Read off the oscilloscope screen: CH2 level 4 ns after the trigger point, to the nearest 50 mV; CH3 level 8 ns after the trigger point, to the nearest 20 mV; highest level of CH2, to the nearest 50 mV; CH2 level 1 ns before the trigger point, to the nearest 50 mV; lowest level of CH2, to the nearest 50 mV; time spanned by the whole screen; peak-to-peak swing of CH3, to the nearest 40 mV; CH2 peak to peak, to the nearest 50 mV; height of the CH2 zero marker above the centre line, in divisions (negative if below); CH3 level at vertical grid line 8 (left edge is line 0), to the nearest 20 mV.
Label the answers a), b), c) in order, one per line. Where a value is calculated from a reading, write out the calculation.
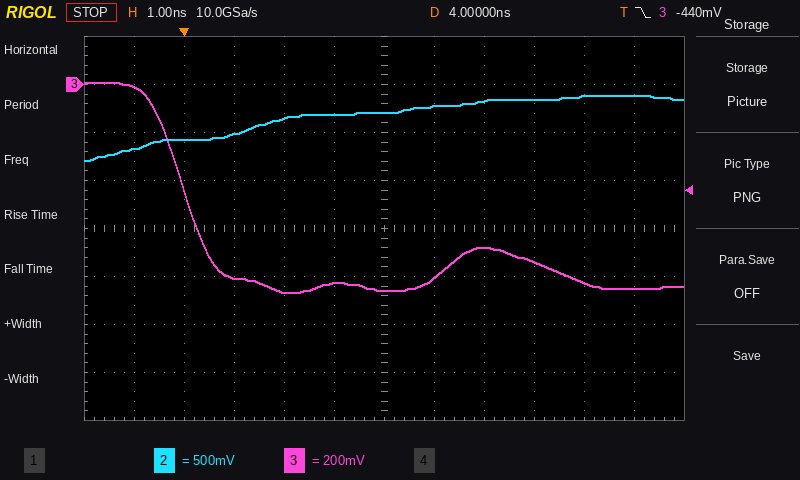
a) -300 mV
b) -820 mV
c) -100 mV
d) -650 mV
e) -800 mV
f) 12 ns
g) 880 mV
h) -100 mV − (-800 mV) = 700 mV
i) +3.0 div
j) -680 mV
